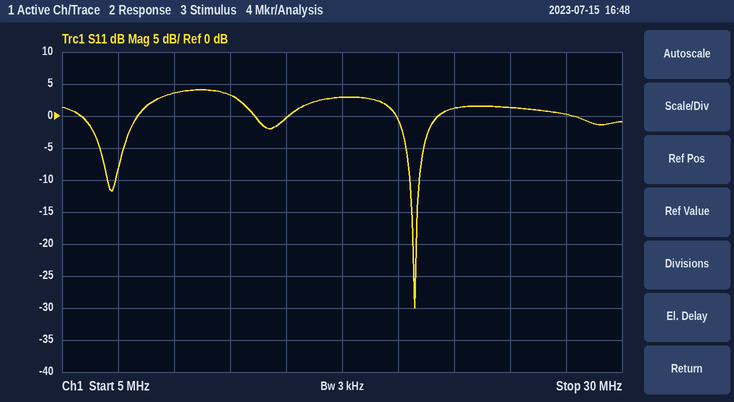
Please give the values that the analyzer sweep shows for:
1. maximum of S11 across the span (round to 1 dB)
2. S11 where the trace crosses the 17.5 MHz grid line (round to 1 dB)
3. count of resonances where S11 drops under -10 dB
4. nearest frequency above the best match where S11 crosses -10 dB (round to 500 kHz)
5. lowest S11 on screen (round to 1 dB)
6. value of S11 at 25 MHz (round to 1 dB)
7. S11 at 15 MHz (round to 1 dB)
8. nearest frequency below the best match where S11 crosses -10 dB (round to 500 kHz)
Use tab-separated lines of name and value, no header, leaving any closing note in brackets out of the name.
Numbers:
maximum of S11 across the span	4 dB
S11 where the trace crosses the 17.5 MHz grid line	3 dB
count of resonances where S11 drops under -10 dB	2
nearest frequency above the best match where S11 crosses -10 dB	21.0 MHz
lowest S11 on screen	-30 dB
value of S11 at 25 MHz	1 dB
S11 at 15 MHz	0 dB
nearest frequency below the best match where S11 crosses -10 dB	20.5 MHz
